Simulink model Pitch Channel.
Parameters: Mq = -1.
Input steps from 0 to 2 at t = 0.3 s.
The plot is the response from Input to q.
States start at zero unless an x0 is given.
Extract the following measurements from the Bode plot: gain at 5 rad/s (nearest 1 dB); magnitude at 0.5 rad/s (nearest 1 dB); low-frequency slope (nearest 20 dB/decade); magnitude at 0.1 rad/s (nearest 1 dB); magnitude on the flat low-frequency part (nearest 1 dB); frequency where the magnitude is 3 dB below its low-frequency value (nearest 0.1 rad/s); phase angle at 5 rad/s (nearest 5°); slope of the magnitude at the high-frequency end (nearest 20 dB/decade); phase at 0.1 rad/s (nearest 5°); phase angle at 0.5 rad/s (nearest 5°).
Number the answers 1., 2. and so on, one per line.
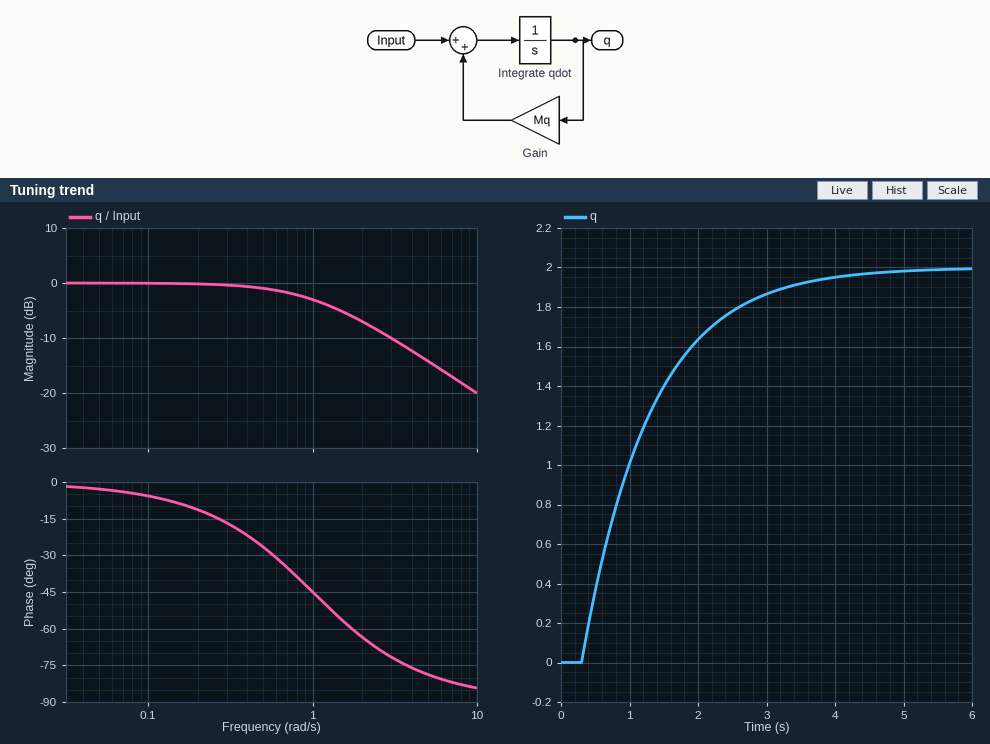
1. -14 dB
2. -1 dB
3. 0 dB/decade
4. 0 dB
5. 0 dB
6. 1.0 rad/s
7. -80°
8. -20 dB/decade
9. -5°
10. -25°
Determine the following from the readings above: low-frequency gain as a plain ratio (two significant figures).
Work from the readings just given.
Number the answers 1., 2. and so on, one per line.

1. 1.0
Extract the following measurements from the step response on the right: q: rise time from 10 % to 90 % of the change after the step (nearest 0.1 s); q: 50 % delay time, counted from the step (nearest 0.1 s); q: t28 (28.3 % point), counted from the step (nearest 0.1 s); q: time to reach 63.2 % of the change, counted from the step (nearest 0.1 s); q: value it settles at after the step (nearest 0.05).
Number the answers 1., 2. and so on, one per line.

1. 2.2 s
2. 0.7 s
3. 0.3 s
4. 1.0 s
5. 2.00
